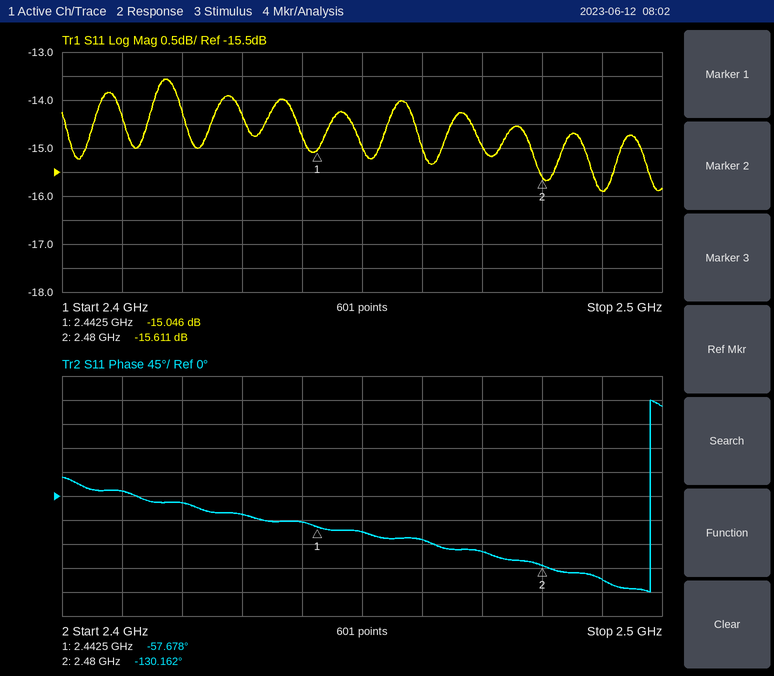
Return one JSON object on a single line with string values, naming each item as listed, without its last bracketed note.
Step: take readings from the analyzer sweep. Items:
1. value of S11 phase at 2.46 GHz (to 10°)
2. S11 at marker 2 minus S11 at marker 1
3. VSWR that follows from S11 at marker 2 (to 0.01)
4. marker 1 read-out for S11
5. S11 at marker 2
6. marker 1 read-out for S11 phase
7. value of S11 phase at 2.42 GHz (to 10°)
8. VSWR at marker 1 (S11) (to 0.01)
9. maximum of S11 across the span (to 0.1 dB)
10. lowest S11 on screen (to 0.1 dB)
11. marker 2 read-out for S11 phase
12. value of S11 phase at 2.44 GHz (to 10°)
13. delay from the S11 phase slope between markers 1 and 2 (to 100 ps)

{"value of S11 phase at 2.46 GHz": "-80°", "S11 at marker 2 minus S11 at marker 1": "-0.565 dB", "VSWR that follows from S11 at marker 2": "1.40", "marker 1 read-out for S11": "-15.046 dB", "S11 at marker 2": "-15.611 dB", "marker 1 read-out for S11 phase": "-57.678°", "value of S11 phase at 2.42 GHz": "-10°", "VSWR at marker 1 (S11)": "1.43", "maximum of S11 across the span": "-13.6 dB", "lowest S11 on screen": "-15.9 dB", "marker 2 read-out for S11 phase": "-130.162°", "value of S11 phase at 2.44 GHz": "-50°", "delay from the S11 phase slope between markers 1 and 2": "5.4 ns"}
